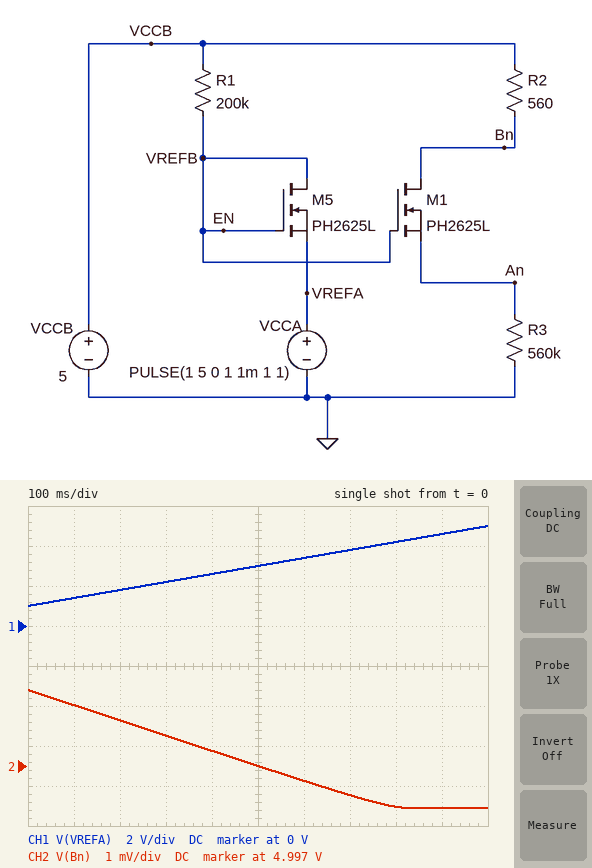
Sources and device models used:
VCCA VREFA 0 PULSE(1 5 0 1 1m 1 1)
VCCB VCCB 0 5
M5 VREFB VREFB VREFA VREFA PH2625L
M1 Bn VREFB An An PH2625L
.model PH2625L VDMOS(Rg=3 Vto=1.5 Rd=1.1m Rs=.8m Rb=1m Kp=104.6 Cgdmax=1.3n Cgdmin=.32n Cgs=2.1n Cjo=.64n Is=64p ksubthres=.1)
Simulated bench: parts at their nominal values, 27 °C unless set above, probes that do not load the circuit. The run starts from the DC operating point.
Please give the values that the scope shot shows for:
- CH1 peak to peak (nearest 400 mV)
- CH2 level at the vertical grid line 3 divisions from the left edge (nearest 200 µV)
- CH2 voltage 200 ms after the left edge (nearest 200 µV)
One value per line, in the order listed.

4.0 V
4.9978 V
4.9982 V
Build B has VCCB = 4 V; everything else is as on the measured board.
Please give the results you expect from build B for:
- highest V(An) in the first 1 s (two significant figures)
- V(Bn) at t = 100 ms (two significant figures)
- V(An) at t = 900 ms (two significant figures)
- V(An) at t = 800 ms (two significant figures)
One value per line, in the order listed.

3.8 V
4.0 V
3.4 V
3.1 V
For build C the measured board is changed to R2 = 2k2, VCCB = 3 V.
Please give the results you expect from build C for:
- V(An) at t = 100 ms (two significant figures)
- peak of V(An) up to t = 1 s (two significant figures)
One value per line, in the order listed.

1.4 V
3.0 V
